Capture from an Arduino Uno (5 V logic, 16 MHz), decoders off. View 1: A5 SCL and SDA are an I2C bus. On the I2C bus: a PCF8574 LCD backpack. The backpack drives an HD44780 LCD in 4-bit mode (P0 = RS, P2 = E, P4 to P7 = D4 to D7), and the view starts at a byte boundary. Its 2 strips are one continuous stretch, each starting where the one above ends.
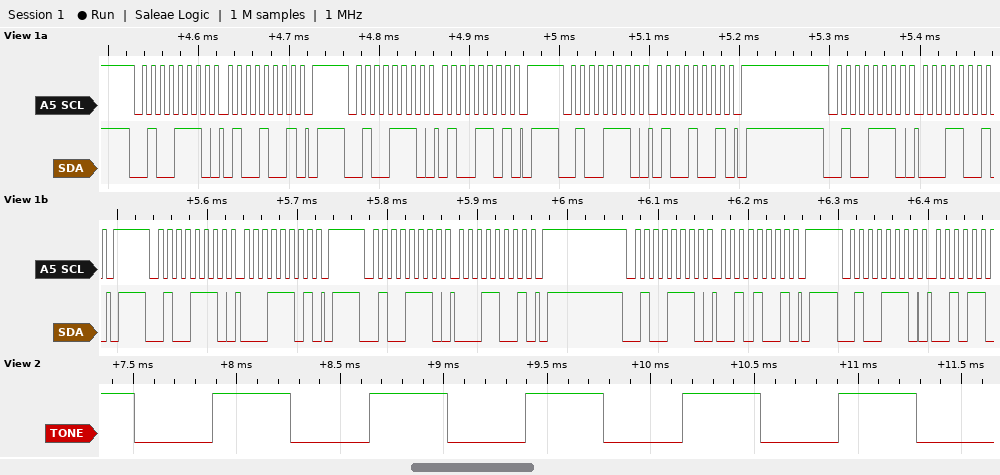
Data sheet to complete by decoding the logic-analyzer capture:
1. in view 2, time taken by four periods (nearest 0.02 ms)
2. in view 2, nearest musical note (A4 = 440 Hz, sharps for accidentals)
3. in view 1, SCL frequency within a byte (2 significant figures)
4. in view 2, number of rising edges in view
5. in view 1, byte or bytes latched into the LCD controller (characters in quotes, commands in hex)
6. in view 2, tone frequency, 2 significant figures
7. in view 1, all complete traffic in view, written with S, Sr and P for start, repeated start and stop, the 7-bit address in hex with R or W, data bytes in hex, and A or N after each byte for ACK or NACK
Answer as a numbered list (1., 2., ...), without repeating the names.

1. 3.02 ms
2. E6
3. 100 kHz
4. 5
5. 'A'
6. 1.3 kHz
7. S 27W A 49 A P S 27W A 4D A P S 27W A 49 A P S 27W A 19 A P S 27W A 1D A P S 27W A 19 A P S 27W A 29 A P S 27W A
